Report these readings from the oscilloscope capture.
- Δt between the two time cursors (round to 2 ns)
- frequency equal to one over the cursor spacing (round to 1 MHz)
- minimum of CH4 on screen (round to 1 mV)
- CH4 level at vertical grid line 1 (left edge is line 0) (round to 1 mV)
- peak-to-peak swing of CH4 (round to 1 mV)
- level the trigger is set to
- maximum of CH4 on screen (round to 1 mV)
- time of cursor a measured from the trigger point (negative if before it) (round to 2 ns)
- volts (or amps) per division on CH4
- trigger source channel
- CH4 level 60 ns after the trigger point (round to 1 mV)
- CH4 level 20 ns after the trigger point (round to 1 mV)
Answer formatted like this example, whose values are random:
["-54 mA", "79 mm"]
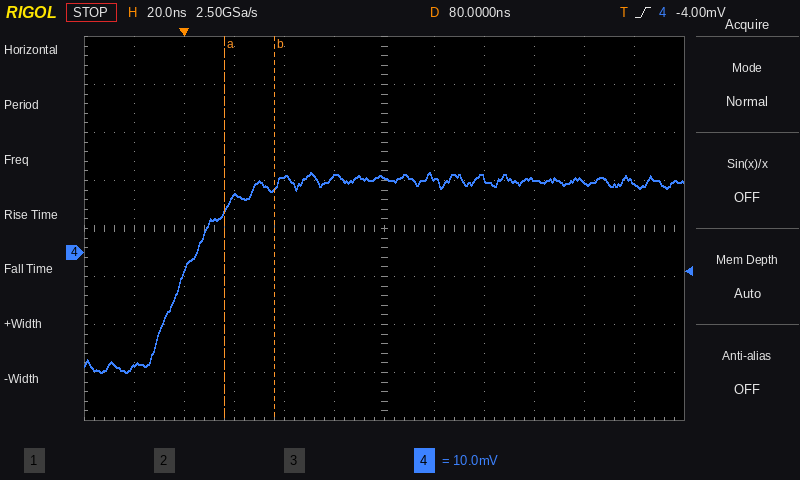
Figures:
["20 ns", "50 MHz", "-25 mV", "-24 mV", "42 mV", "-4.00 mV", "17 mV", "+16 ns", "10 mV", "CH4", "16 mV", "12 mV"]
